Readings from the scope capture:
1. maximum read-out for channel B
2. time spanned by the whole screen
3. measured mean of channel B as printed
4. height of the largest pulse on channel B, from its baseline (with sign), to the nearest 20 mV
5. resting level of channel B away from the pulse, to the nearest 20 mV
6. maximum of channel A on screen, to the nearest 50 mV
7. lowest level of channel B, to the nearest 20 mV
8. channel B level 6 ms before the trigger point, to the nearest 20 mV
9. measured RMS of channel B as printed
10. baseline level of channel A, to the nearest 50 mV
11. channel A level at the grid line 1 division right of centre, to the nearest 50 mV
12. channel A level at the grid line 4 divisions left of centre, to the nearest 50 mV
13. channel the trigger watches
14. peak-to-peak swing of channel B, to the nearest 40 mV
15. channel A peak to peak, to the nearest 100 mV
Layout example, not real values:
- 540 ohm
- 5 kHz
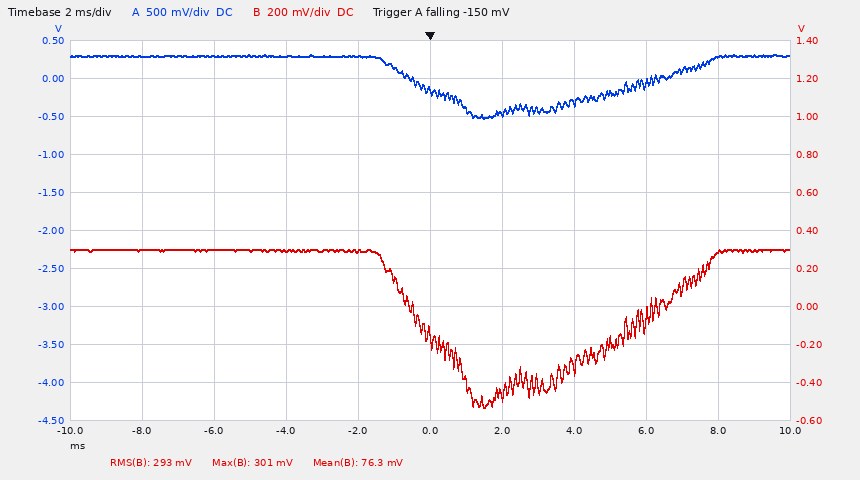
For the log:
- 301 mV
- 20 ms
- 76.3 mV
- -840 mV
- 300 mV
- 300 mV
- -540 mV
- 300 mV
- 293 mV
- 300 mV
- -450 mV
- 300 mV
- channel A
- 840 mV
- 800 mV
